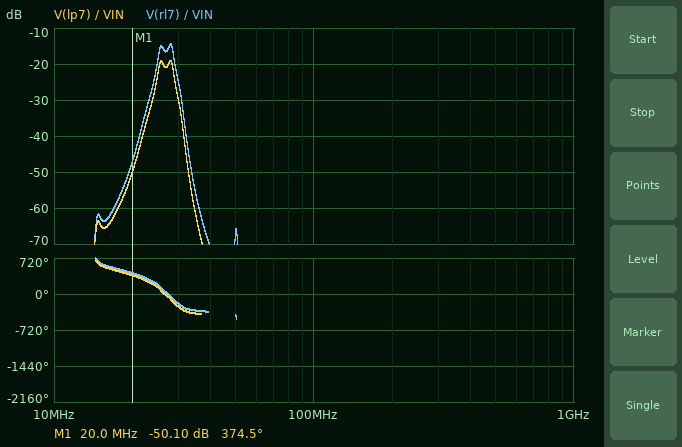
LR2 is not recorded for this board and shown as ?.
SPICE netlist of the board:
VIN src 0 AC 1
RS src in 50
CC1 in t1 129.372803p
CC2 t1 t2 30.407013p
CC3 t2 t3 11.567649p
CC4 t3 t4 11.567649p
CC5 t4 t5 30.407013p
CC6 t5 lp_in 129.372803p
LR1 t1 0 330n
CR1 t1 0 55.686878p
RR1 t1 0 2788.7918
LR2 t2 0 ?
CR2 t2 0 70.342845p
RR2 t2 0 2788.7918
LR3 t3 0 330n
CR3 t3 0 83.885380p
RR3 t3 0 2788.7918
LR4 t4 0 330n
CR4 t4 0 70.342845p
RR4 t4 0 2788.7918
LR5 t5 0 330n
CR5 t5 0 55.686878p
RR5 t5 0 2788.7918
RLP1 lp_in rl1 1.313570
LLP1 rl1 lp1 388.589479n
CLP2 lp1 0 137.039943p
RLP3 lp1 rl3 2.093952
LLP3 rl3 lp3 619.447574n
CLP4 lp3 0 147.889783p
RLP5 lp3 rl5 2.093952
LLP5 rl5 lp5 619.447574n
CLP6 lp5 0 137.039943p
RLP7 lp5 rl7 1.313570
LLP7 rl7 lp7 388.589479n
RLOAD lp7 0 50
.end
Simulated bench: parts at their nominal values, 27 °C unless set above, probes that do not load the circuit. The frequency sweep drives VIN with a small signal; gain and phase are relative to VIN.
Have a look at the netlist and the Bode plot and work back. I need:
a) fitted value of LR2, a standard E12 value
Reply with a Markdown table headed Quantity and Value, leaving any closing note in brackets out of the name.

| Quantity | Value |
|---|---|
| fitted value of LR2, a standard E12 value | 1 µH |
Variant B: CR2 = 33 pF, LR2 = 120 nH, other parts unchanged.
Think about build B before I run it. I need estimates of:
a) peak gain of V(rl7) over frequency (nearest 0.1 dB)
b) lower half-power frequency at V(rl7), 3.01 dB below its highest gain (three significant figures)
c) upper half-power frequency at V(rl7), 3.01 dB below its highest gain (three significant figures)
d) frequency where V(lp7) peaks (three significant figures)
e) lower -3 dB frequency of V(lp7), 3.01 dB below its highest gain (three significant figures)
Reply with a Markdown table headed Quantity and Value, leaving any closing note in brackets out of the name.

| Quantity | Value |
|---|---|
| peak gain of V(rl7) over frequency | -23.3 dB |
| lower half-power frequency at V(rl7), 3.01 dB below its highest gain | 25.4 MHz |
| upper half-power frequency at V(rl7), 3.01 dB below its highest gain | 28.7 MHz |
| frequency where V(lp7) peaks | 27.9 MHz |
| lower -3 dB frequency of V(lp7), 3.01 dB below its highest gain | 25.3 MHz |
